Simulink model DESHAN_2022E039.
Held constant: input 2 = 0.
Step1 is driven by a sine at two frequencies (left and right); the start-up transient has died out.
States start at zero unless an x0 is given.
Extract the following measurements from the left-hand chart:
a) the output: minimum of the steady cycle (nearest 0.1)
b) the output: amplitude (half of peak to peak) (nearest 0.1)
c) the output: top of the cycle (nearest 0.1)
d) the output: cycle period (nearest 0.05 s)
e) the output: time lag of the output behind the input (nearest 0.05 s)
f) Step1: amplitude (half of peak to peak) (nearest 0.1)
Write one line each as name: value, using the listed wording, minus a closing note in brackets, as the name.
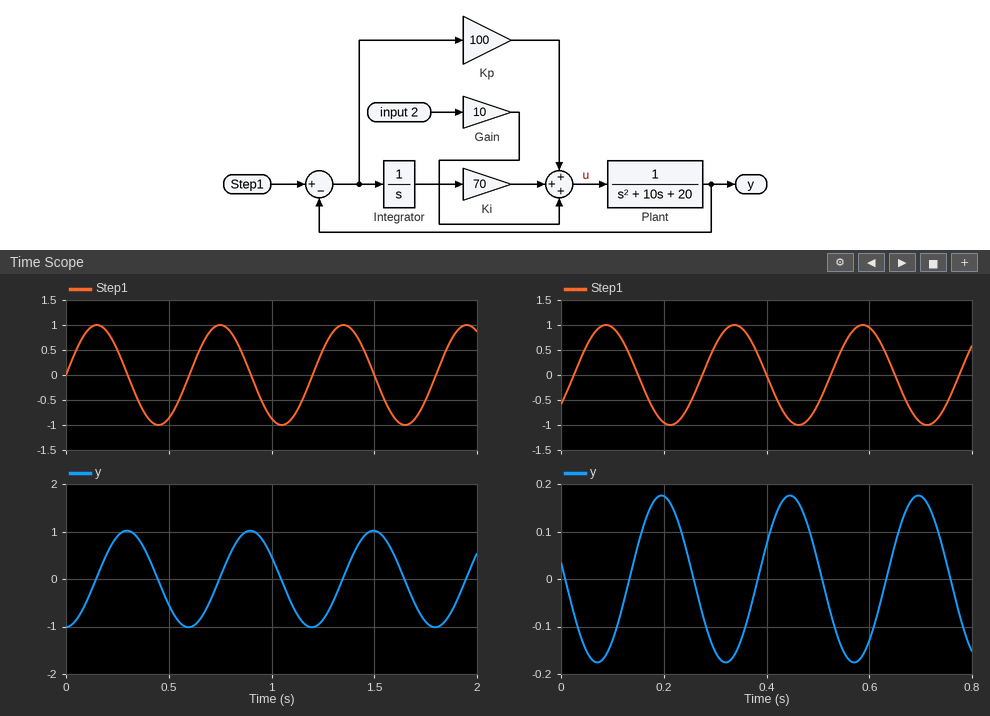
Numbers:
the output: minimum of the steady cycle: -1.0
the output: amplitude (half of peak to peak): 1.0
the output: top of the cycle: 1.0
the output: cycle period: 0.60 s
the output: time lag of the output behind the input: 0.15 s
Step1: amplitude (half of peak to peak): 1.0
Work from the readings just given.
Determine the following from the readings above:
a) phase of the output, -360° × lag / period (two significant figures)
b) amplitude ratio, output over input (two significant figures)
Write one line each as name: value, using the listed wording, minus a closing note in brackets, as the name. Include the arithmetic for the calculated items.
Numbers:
phase of the output, -360° × lag / period: -360 × 0.15 / 0.6 = -90°
amplitude ratio, output over input: 1 / 1 = 1.0
